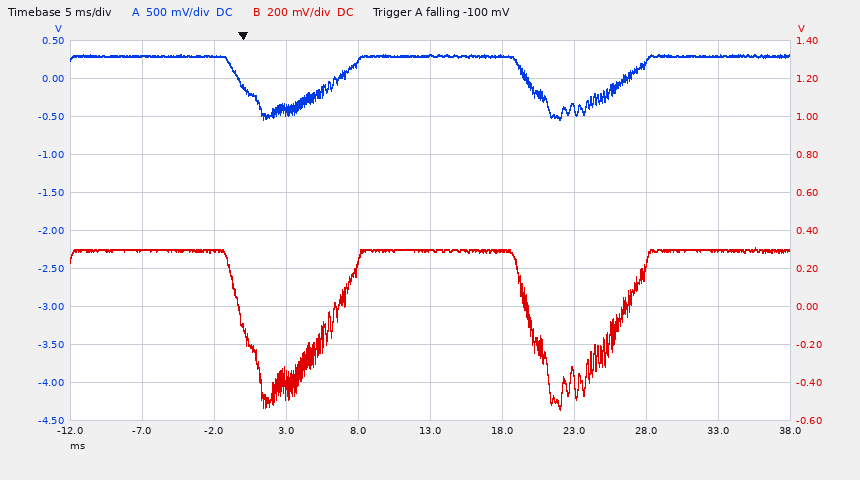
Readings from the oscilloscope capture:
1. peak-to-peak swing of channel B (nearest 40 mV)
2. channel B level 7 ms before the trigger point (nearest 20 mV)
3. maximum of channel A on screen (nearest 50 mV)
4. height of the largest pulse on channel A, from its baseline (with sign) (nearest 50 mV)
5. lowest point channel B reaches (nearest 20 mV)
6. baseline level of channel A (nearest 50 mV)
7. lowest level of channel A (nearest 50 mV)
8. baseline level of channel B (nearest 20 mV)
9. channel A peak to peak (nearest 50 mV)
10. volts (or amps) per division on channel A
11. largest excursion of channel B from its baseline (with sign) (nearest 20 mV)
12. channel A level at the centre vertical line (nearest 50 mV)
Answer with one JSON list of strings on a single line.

["840 mV", "300 mV", "300 mV", "-850 mV", "-540 mV", "300 mV", "-550 mV", "300 mV", "850 mV", "500 mV", "-840 mV", "300 mV"]
